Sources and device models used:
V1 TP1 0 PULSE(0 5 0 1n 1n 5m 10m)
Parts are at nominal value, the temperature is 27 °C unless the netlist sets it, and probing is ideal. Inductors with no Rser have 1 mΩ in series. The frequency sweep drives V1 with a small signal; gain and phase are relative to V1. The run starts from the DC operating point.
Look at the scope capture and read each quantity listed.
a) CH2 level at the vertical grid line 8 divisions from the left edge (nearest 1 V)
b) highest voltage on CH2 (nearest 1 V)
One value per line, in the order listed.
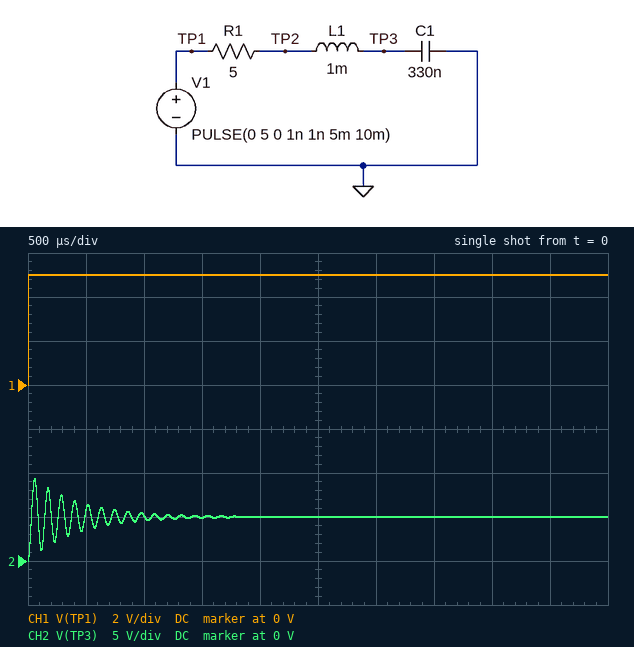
5 V
9 V
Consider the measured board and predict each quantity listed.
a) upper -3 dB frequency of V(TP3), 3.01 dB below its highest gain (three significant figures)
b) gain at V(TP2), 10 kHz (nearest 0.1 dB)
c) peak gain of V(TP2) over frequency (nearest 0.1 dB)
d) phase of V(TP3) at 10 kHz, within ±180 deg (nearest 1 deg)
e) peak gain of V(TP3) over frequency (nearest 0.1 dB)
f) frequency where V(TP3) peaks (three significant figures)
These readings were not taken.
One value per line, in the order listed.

9.13 kHz
-0.5 dB
0 dB
-161 deg
20.8 dB
8.74 kHz
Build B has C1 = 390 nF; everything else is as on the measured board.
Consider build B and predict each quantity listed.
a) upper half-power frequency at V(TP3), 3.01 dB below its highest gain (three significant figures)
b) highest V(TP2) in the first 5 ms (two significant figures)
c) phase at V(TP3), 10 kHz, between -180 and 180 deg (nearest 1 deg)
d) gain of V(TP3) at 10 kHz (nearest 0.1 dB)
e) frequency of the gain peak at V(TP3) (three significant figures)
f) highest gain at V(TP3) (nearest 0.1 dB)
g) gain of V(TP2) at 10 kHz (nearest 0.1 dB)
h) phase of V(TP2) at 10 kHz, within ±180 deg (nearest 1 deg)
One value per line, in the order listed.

8.43 kHz
5.4 V
-167 deg
5.1 dB
8.04 kHz
20.1 dB
-0.2 dB
13 deg
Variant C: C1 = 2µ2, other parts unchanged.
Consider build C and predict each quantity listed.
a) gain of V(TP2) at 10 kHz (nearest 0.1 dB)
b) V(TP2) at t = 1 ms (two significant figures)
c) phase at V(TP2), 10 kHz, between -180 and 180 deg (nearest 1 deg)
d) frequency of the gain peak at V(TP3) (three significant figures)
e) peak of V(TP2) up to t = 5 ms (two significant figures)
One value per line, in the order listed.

0 dB
4.9 V
5 deg
3.35 kHz
5.7 V
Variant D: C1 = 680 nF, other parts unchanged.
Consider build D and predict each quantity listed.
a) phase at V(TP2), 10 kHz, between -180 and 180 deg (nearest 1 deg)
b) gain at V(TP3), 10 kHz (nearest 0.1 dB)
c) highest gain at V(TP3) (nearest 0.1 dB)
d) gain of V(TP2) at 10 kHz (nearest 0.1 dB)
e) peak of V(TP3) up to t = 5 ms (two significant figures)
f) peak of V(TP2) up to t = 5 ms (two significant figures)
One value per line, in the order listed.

7 deg
-4.6 dB
17.7 dB
-0.1 dB
9.1 V
5.5 V
